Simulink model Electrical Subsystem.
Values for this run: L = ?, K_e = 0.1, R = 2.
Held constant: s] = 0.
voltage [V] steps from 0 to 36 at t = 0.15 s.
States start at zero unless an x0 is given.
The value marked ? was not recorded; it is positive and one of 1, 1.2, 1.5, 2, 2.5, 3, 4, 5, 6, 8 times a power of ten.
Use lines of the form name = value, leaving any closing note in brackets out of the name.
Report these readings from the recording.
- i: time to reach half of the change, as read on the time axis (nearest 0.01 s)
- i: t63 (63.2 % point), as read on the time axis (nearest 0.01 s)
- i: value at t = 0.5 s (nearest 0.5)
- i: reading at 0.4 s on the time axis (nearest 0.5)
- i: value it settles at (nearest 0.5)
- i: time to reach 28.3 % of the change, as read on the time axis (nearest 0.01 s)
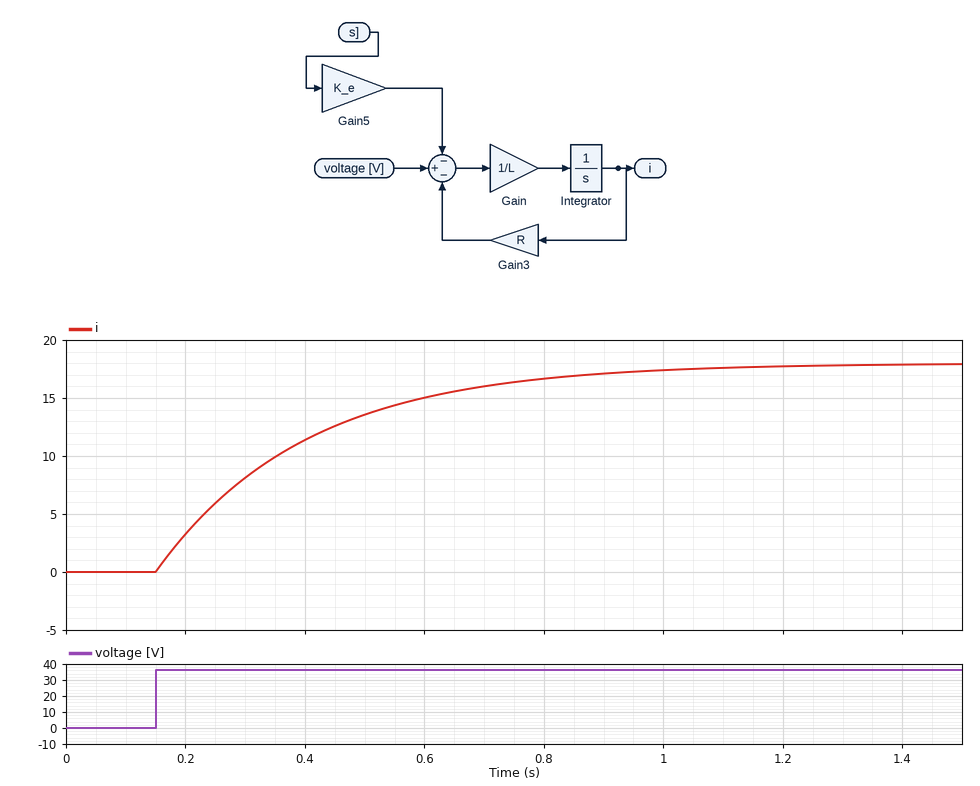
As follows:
i: time to reach half of the change, as read on the time axis = 0.32 s
i: t63 (63.2 % point), as read on the time axis = 0.40 s
i: value at t = 0.5 s = 13.5
i: reading at 0.4 s on the time axis = 11.5
i: value it settles at = 18.0
i: time to reach 28.3 % of the change, as read on the time axis = 0.23 s
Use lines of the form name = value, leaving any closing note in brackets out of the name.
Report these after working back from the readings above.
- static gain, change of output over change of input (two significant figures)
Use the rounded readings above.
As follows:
static gain, change of output over change of input = 0.50
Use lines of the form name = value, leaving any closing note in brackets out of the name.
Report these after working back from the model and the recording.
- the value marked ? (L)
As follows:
the value marked ? = 0.5
